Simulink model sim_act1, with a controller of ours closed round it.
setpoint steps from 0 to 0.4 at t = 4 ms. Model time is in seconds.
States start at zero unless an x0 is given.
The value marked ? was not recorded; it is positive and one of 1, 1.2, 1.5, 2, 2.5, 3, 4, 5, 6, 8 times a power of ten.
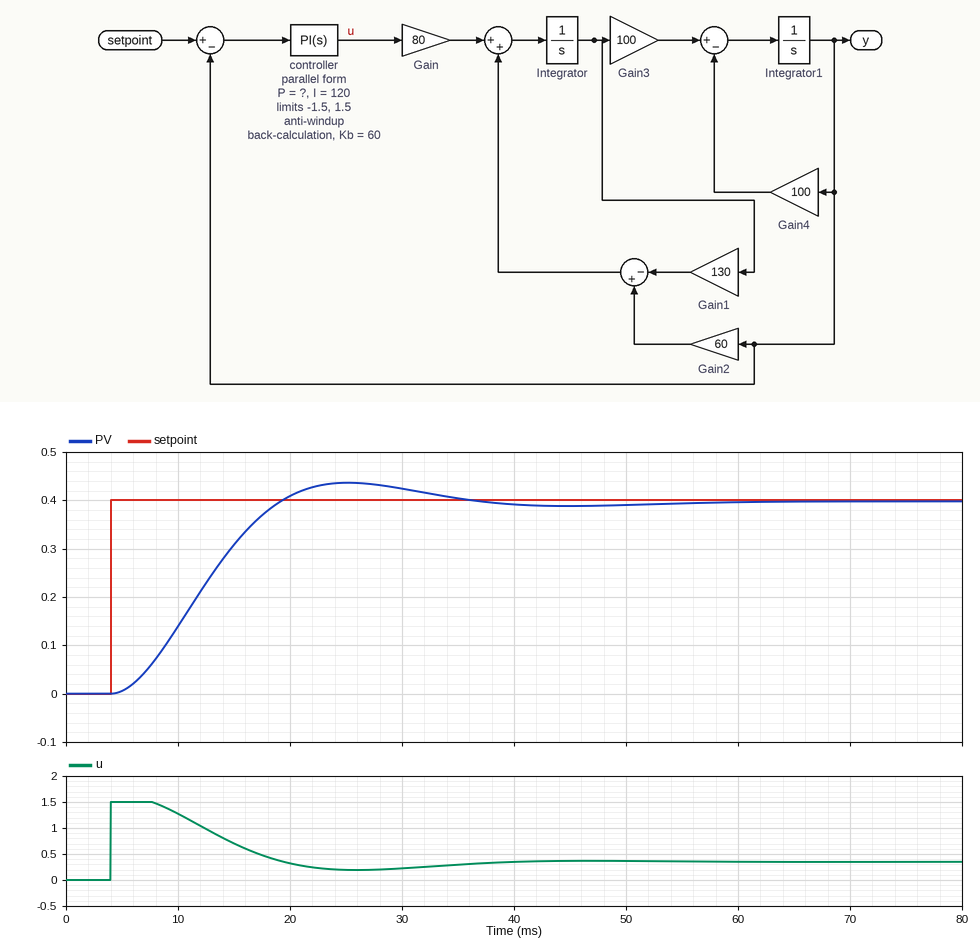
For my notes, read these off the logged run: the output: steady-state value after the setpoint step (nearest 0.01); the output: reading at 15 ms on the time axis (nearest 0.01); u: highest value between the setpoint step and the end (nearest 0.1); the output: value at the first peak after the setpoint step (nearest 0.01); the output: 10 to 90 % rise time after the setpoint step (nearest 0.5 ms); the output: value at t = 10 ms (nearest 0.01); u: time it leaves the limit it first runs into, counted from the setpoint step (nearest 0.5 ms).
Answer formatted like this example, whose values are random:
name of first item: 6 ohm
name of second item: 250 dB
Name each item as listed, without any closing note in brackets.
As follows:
the output: steady-state value after the setpoint step: 0.40
the output: reading at 15 ms on the time axis: 0.31
u: highest value between the setpoint step and the end: 1.5
the output: value at the first peak after the setpoint step: 0.44
the output: 10 to 90 % rise time after the setpoint step: 10.0 ms
the output: value at t = 10 ms: 0.14
u: time it leaves the limit it first runs into, counted from the setpoint step: 4.0 ms
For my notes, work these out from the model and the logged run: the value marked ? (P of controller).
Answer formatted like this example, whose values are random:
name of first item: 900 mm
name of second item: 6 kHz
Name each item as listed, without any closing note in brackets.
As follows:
the value marked ?: 4
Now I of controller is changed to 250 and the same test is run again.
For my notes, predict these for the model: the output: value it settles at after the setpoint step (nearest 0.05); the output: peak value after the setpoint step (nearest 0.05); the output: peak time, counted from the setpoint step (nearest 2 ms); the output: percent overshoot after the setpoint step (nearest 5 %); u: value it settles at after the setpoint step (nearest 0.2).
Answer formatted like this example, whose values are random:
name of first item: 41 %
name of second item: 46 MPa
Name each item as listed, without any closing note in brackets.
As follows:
the output: value it settles at after the setpoint step: 0.40
the output: peak value after the setpoint step: 0.50
the output: peak time, counted from the setpoint step: 22 ms
the output: percent overshoot after the setpoint step: 25 %
u: value it settles at after the setpoint step: 0.4
